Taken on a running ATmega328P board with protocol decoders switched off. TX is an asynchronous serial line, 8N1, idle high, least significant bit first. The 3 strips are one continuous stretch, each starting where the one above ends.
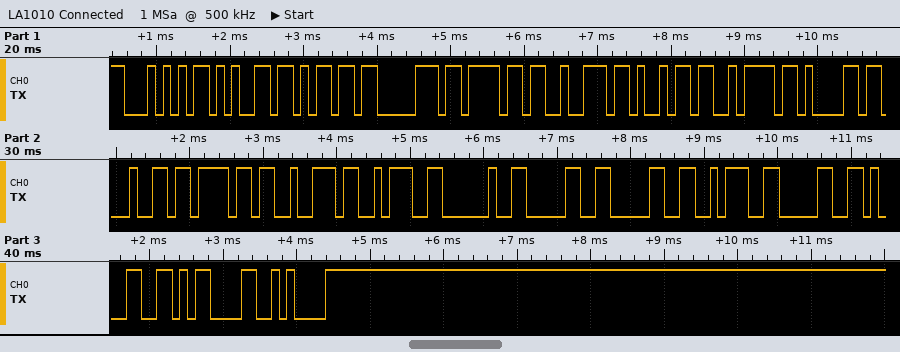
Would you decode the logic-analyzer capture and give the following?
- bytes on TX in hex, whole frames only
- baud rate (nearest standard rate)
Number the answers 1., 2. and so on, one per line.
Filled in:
1. 54 65 6D 70 6F 72 69 7A 61 64 6F 72 3A 20 30 30 3A 30 31 0D 0A
2. 9600 baud
